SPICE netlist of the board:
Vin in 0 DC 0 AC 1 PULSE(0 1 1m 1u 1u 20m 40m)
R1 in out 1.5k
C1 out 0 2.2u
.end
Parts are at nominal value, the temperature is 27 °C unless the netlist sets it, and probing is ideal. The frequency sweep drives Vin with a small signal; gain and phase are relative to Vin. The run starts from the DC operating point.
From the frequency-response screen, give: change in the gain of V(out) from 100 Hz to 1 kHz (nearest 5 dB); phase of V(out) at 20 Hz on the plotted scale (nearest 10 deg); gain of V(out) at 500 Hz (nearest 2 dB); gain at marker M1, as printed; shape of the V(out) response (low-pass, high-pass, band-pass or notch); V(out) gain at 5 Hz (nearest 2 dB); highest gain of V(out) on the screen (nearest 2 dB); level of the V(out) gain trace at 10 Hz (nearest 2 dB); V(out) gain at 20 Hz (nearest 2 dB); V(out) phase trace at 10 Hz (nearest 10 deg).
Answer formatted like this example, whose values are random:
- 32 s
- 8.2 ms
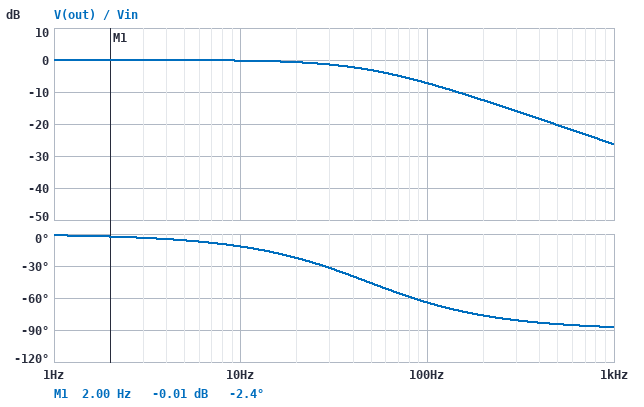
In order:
- -20 dB
- -20 deg
- -20 dB
- -0.01 dB
- low-pass
- 0 dB
- 0 dB
- 0 dB
- 0 dB
- -10 deg
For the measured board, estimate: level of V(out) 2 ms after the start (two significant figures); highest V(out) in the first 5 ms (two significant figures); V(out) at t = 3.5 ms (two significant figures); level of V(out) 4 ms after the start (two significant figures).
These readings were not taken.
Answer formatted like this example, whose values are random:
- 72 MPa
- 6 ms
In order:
- 260 mV
- 700 mV
- 530 mV
- 600 mV
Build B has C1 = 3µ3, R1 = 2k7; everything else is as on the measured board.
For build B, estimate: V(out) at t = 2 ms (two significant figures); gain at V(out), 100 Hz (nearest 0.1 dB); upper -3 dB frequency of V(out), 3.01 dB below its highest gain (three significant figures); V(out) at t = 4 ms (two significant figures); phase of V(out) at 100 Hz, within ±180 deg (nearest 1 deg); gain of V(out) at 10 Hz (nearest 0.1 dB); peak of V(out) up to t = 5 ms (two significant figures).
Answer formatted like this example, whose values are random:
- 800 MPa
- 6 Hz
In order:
- 110 mV
- -15.1 dB
- 17.9 Hz
- 290 mV
- -80 deg
- -1.2 dB
- 360 mV
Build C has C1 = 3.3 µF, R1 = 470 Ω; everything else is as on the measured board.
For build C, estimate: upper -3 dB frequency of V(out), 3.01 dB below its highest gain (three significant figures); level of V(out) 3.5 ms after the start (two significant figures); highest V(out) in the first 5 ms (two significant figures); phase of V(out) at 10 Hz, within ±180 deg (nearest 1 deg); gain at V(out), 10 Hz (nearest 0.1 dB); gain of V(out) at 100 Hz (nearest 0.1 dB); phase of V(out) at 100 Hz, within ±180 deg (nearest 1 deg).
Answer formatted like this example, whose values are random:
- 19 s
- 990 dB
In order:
- 103 Hz
- 800 mV
- 920 mV
- -6 deg
- 0 dB
- -2.9 dB
- -44 deg
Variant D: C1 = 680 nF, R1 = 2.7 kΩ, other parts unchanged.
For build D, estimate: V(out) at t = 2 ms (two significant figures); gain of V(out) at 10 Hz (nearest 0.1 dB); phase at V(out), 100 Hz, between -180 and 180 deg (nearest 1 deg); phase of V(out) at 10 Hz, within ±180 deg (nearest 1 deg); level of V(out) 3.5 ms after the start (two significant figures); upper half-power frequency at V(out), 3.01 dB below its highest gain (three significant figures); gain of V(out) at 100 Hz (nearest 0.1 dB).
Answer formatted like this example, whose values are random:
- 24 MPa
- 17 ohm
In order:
- 420 mV
- -0.1 dB
- -49 deg
- -7 deg
- 740 mV
- 86.7 Hz
- -3.7 dB
